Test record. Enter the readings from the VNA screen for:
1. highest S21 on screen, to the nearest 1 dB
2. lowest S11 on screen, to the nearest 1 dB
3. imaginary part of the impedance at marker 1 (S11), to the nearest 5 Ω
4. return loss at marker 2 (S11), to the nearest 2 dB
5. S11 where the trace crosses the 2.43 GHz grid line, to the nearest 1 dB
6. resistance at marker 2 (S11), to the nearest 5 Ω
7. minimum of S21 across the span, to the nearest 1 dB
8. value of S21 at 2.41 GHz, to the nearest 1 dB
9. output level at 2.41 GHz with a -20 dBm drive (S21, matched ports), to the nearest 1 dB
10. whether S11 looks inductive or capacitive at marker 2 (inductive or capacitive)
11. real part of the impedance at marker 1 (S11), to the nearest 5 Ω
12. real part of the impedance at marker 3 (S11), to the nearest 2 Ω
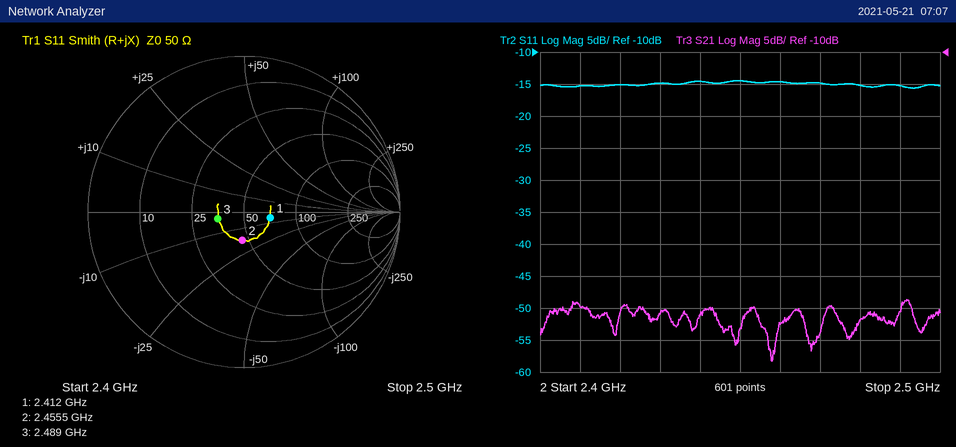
-49 dB
-16 dB
-5 Ω
14 dB
-15 dB
45 Ω
-58 dB
-50 dB
-70 dBm
capacitive
70 Ω
36 Ω
